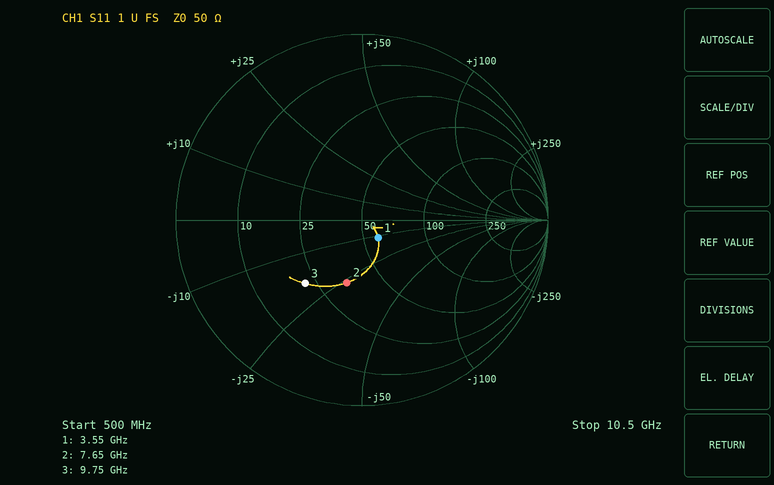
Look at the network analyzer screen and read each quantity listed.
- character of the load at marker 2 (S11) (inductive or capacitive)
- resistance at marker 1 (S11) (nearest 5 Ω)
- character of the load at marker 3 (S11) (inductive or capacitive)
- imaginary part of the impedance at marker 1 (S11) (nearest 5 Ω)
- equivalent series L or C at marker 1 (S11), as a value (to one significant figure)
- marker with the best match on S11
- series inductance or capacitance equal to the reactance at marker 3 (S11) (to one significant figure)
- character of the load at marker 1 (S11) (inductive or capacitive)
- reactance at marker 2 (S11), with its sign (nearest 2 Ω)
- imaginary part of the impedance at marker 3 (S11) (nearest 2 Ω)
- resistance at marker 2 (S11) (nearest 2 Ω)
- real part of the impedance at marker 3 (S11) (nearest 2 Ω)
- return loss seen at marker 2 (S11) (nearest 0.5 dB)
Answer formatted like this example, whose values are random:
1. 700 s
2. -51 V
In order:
1. capacitive
2. 60 Ω
3. capacitive
4. -10 Ω
5. 4 pF
6. marker 1
7. 900 fF
8. capacitive
9. -26 Ω
10. -18 Ω
11. 34 Ω
12. 22 Ω
13. 9.0 dB
